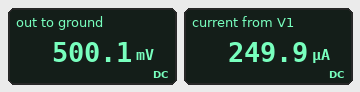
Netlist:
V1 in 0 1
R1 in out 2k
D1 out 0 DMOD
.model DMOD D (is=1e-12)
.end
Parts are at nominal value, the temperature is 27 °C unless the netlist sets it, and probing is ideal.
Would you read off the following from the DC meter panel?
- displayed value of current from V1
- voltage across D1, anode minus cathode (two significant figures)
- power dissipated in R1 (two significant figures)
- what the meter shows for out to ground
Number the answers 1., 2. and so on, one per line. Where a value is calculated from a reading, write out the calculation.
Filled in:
1. 249.9 µA
2. 500.1 mV = 500 mV
3. (1 V - 500.1 mV)^2 / 2 kΩ = 120 µW
4. 500.1 mV
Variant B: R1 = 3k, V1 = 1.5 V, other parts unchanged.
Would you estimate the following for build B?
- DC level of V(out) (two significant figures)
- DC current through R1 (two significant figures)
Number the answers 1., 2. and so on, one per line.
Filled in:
1. 510 mV
2. 330 µA
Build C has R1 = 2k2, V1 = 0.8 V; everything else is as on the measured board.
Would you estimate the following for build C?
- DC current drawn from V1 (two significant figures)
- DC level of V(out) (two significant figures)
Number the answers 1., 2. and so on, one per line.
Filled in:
1. 140 µA
2. 490 mV
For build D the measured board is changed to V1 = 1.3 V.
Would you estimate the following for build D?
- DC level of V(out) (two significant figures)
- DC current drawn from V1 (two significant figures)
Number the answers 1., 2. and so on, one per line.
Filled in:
1. 510 mV
2. 390 µA
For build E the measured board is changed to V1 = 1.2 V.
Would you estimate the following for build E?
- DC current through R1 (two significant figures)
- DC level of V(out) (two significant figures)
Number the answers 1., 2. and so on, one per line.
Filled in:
1. 350 µA
2. 510 mV
